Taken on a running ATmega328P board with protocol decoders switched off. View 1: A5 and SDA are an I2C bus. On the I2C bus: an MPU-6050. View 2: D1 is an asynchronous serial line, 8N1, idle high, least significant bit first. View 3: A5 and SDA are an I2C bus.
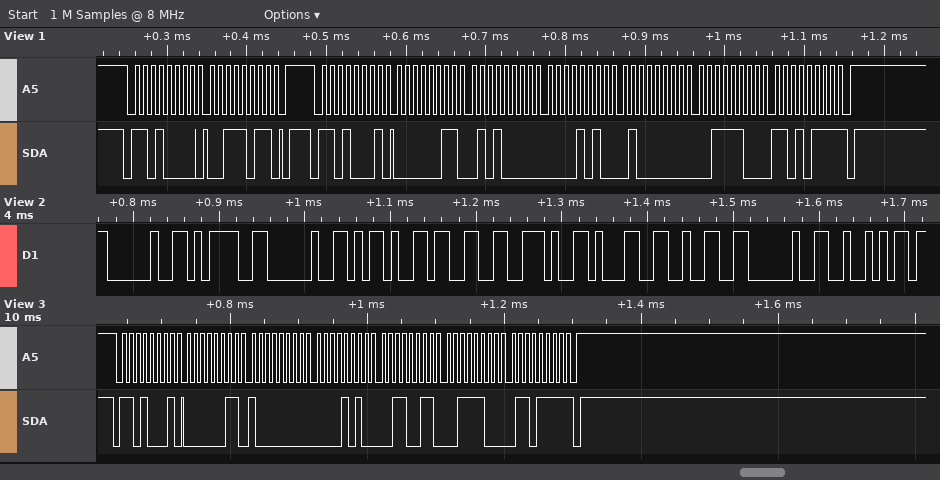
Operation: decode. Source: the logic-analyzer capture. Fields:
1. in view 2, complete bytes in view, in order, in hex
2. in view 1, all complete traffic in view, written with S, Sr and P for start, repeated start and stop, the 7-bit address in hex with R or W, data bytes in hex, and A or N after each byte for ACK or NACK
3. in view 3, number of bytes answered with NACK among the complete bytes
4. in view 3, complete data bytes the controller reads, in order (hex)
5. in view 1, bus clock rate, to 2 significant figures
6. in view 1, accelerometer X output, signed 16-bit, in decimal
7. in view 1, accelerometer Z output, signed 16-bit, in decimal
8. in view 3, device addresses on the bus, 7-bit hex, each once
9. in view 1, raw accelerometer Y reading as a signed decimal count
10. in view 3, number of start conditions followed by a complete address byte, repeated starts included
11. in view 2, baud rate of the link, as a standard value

20 3D 20 2D 33 2E 31 32 20 52
S 68W A 3B A P S 68R A 03 A 50 A 0A A 40 A 3C A D7 N P
1
03 80 0A 33 3C 6F
100 kHz
848
15575
0x68
2624
1
115200 baud
